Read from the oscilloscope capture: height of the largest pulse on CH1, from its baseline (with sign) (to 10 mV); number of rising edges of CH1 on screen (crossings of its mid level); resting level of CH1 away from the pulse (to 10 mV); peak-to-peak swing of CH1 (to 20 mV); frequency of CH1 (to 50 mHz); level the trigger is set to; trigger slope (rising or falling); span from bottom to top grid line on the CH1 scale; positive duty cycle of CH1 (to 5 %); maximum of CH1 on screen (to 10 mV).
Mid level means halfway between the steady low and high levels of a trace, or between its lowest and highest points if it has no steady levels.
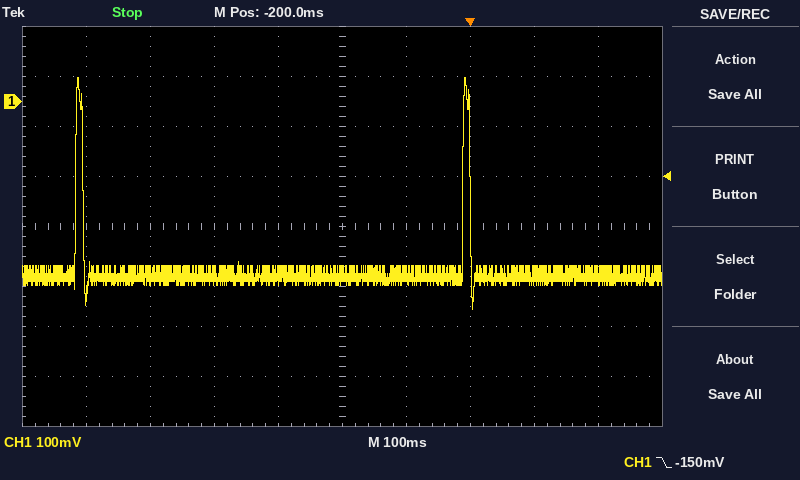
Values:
+400 mV
2
-350 mV
460 mV
1.65 Hz
-150 mV
falling
800 mV
0 %
50 mV
